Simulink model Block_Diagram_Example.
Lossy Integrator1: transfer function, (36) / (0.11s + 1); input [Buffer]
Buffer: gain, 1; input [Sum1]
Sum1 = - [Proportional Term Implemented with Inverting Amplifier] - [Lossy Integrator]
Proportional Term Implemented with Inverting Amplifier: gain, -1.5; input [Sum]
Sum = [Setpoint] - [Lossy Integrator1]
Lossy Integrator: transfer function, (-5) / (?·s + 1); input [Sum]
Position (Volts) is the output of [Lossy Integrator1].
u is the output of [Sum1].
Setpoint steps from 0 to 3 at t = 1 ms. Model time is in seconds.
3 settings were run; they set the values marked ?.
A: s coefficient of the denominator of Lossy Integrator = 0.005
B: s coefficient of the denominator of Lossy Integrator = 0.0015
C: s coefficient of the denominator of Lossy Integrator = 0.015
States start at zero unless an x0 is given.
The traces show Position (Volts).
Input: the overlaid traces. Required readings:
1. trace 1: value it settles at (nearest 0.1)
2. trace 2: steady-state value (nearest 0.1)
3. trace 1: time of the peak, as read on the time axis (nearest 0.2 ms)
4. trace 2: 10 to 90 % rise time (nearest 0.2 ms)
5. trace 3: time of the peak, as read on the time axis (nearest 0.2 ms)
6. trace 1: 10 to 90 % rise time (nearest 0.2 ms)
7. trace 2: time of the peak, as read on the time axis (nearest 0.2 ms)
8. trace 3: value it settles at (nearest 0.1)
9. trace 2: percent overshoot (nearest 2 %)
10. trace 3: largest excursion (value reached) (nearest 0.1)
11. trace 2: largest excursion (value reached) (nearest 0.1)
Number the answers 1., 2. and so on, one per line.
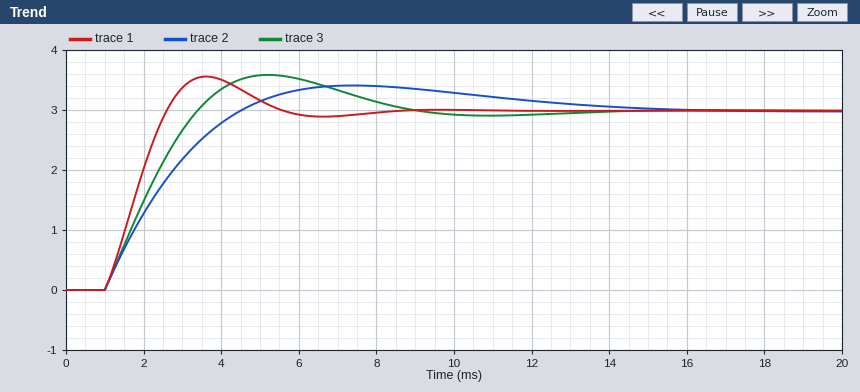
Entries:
1. 3.0
2. 3.0
3. 3.6 ms
4. 2.6 ms
5. 5.2 ms
6. 1.2 ms
7. 7.4 ms
8. 3.0
9. 14 %
10. 3.6
11. 3.4
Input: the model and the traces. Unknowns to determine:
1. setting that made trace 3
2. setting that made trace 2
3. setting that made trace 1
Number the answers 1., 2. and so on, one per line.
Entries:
1. A
2. C
3. B
